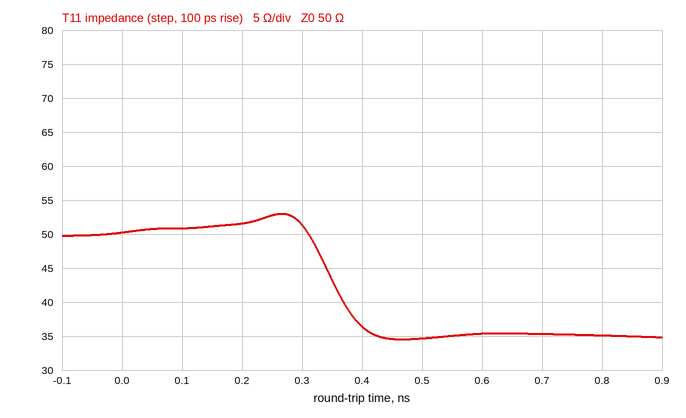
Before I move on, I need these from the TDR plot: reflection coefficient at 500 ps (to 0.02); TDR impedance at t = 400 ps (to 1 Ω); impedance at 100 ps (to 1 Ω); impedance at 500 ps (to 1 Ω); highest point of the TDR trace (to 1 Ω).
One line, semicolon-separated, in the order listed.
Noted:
-0.18; 36 Ω; 51 Ω; 35 Ω; 53 Ω
